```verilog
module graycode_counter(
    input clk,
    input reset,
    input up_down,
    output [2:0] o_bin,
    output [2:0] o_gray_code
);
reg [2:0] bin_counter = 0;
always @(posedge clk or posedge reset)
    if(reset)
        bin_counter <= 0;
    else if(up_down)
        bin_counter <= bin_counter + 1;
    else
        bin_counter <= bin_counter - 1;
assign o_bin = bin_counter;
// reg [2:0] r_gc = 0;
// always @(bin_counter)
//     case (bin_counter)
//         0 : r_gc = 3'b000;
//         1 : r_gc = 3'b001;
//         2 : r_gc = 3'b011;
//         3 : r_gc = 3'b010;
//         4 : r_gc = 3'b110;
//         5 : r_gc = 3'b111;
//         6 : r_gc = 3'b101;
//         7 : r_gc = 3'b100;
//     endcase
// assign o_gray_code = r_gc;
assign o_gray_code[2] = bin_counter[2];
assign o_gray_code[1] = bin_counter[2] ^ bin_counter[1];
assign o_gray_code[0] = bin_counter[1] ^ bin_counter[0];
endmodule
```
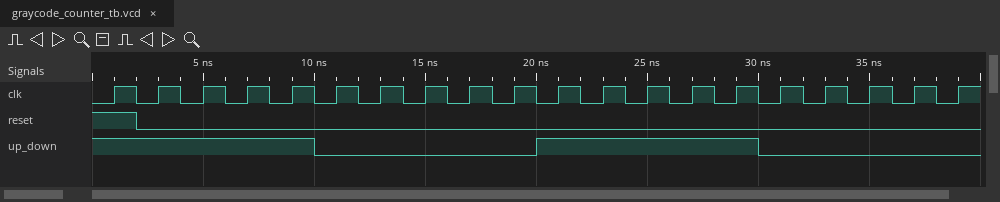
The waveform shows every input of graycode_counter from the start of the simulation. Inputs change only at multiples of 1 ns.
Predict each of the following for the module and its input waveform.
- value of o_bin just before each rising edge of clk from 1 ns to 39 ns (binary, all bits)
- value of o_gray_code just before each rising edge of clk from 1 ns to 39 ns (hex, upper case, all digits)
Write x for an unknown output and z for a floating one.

000, 000, 001, 010, 011, 100, 011, 010, 001, 000, 111, 000, 001, 010, 011, 100, 011, 010, 001, 000
0, 0, 1, 3, 2, 6, 2, 3, 1, 0, 4, 0, 1, 3, 2, 6, 2, 3, 1, 0
